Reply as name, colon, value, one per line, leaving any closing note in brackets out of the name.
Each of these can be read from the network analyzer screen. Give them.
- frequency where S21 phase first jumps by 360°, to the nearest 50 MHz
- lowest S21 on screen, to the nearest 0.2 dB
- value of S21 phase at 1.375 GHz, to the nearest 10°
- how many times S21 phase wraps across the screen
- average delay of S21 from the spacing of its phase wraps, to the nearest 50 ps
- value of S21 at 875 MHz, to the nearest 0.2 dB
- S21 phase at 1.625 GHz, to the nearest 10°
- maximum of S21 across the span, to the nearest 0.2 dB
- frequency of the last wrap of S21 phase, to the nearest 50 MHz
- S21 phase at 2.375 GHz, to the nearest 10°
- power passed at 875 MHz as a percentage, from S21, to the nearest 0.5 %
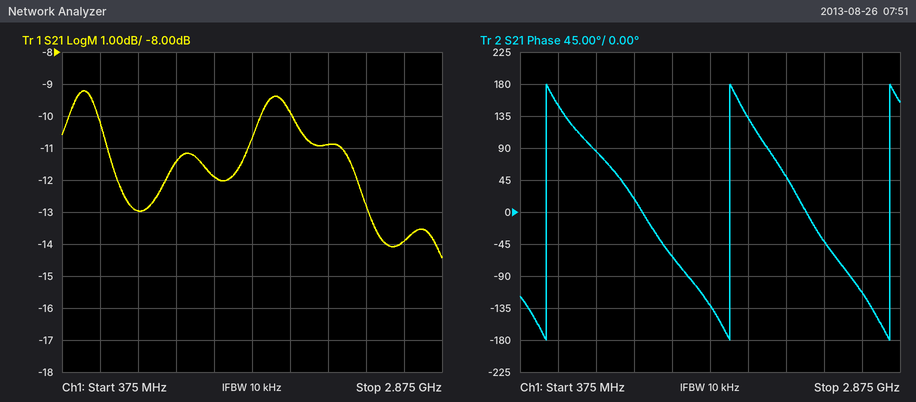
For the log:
frequency where S21 phase first jumps by 360°, to the nearest 50 MHz: 550 MHz
lowest S21 on screen, to the nearest 0.2 dB: -14.4 dB
value of S21 phase at 1.375 GHz, to the nearest 10°: -60°
how many times S21 phase wraps across the screen: 3
average delay of S21 from the spacing of its phase wraps, to the nearest 50 ps: 900 ps
value of S21 at 875 MHz, to the nearest 0.2 dB: -13.0 dB
S21 phase at 1.625 GHz, to the nearest 10°: -130°
maximum of S21 across the span, to the nearest 0.2 dB: -9.2 dB
frequency of the last wrap of S21 phase, to the nearest 50 MHz: 2.80 GHz
S21 phase at 2.375 GHz, to the nearest 10°: -40°
power passed at 875 MHz as a percentage, from S21, to the nearest 0.5 %: 5.0 %
